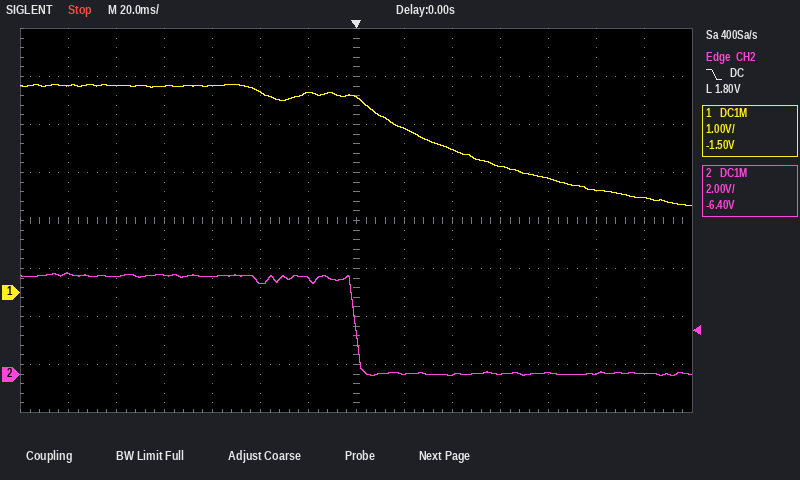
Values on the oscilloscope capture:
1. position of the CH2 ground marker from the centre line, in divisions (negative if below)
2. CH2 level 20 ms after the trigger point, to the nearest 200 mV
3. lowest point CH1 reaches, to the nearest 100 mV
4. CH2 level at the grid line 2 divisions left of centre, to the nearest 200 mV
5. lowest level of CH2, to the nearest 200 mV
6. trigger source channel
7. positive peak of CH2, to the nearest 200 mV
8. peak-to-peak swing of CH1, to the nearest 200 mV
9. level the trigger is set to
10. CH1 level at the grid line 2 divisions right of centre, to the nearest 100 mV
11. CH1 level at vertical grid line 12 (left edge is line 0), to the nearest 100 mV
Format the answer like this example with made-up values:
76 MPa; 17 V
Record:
-3.2 div; 0.0 V; 1.8 V; 3.8 V; 0.0 V; CH2; 4.2 V; 2.6 V; 1.80 V; 3.0 V; 2.1 V
